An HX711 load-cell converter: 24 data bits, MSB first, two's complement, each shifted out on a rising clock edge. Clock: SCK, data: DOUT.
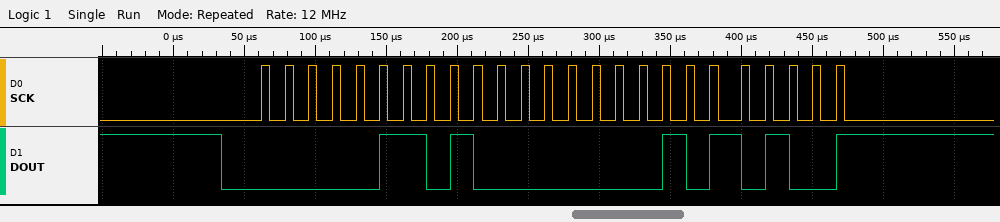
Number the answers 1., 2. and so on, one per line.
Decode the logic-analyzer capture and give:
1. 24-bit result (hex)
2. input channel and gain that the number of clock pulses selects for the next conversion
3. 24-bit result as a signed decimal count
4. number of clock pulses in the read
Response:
1. 0x068054
2. channel A, gain 128
3. 426068
4. 25
